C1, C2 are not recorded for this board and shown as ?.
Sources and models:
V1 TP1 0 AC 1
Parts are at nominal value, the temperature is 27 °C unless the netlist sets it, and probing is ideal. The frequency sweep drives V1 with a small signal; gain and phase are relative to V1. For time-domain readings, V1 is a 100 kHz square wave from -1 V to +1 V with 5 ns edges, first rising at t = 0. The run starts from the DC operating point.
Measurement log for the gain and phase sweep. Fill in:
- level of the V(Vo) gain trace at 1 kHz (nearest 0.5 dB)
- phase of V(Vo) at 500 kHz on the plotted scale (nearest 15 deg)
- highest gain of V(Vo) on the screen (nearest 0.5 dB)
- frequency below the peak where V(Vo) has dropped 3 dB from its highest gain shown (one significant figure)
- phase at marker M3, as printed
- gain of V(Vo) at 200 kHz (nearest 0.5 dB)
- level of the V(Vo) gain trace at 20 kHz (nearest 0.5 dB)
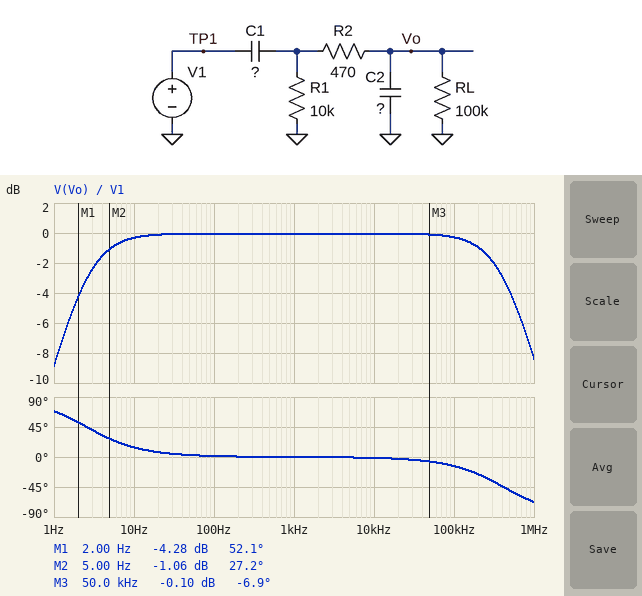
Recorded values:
0 dB
-45 deg
0 dB
3 Hz
-6.9 deg
-1.0 dB
0 dB
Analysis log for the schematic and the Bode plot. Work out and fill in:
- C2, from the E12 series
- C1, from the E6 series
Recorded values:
820 pF
6.8 µF
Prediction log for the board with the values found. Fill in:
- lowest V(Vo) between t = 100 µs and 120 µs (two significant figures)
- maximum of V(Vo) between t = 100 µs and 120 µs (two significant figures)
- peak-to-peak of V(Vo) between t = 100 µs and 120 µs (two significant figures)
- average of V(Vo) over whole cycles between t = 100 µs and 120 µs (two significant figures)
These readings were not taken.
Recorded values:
-1.9 mV
2.0 V
2.0 V
990 mV
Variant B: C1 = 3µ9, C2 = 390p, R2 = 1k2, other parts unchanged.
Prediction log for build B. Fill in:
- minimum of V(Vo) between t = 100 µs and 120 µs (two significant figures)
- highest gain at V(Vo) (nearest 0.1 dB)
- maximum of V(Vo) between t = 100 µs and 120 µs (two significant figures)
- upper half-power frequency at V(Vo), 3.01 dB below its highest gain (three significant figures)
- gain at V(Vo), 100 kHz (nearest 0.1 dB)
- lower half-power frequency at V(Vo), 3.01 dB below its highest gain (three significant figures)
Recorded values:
-3.3 mV
-0.1 dB
2.0 V
344 kHz
-0.5 dB
4.48 Hz
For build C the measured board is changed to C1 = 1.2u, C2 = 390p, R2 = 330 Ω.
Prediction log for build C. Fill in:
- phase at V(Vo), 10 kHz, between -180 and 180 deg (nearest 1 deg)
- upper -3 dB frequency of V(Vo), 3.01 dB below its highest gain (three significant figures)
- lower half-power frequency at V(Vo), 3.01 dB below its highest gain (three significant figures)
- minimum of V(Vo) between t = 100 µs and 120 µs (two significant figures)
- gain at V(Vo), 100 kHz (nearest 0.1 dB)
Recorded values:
0 deg
1.24 MHz
14.6 Hz
-11 mV
-0.1 dB
